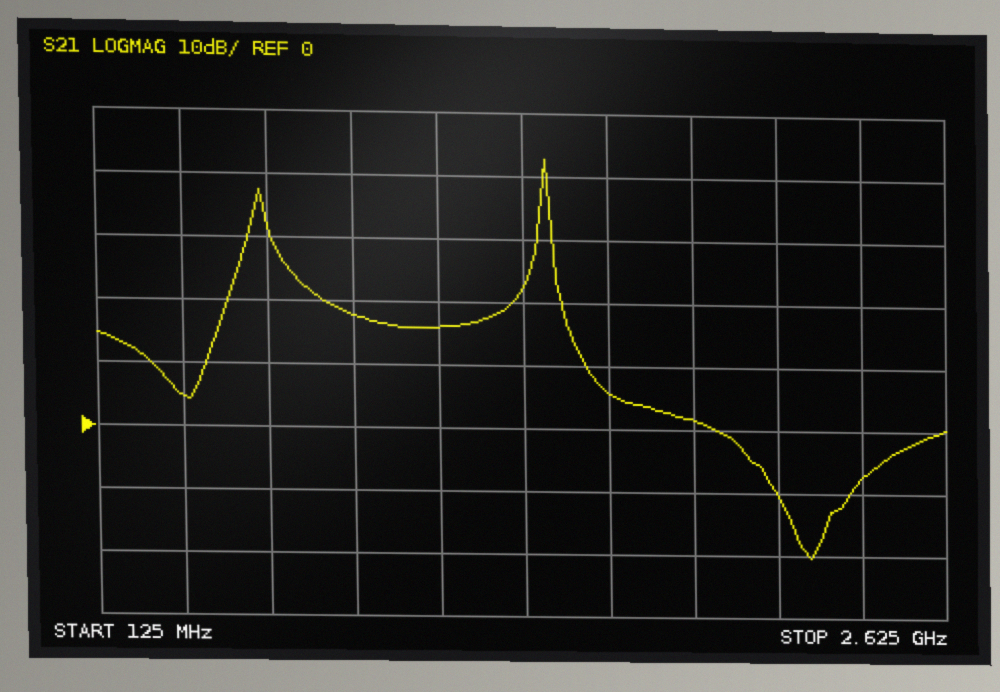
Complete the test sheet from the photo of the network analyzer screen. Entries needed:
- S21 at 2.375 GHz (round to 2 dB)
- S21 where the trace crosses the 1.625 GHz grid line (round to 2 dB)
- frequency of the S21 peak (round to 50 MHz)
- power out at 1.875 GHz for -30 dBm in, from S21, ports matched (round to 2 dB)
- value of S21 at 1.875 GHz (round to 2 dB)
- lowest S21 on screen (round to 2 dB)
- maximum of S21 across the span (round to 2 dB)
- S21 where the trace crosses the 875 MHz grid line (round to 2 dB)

-8 dB
6 dB
1.45 GHz
-28 dBm
2 dB
-20 dB
42 dB
18 dB
